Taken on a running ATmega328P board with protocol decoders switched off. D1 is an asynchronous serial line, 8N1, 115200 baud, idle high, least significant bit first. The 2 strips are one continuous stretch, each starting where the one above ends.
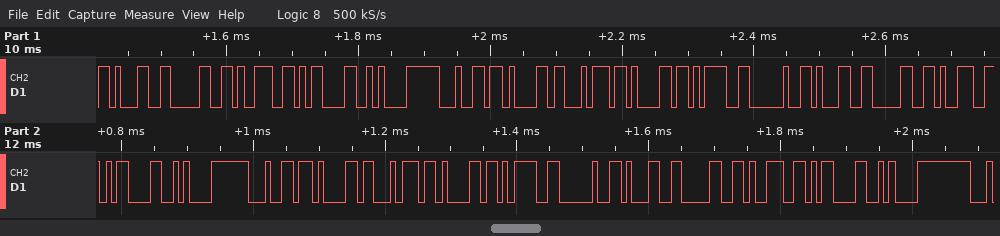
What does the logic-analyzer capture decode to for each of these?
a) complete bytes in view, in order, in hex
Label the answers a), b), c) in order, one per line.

a) 0x31 0x30 0x39 0x0D 0x0A 0x64 0x61 0x74 0x61 0x3D 0x20 0x31 0x30 0x39 0x0D 0x0A 0x64 0x61 0x74 0x61 0x3D 0x20 0x31 0x30 0x39 0x0D 0x0A
